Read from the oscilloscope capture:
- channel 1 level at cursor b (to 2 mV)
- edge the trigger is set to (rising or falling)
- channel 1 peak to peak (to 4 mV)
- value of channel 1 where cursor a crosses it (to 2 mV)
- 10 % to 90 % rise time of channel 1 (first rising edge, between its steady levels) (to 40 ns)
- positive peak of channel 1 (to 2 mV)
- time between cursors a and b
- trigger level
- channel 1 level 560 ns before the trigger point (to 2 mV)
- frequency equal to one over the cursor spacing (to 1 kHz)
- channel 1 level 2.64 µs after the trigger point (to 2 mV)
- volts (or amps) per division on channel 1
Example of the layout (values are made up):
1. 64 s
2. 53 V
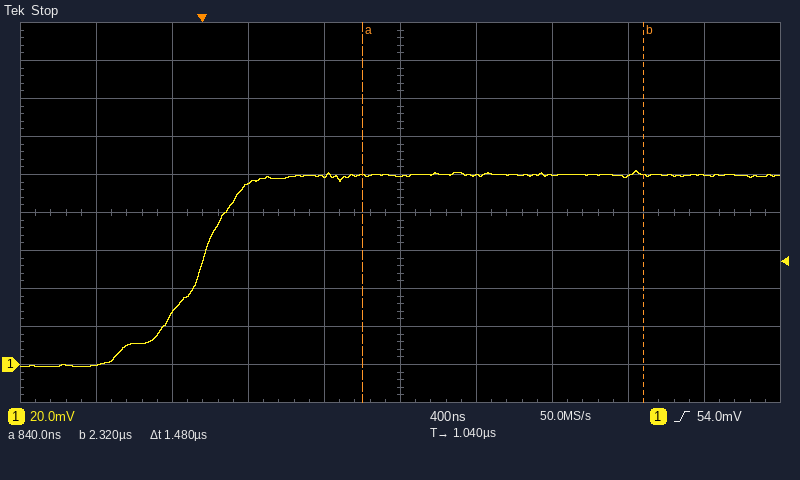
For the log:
1. 100 mV
2. rising
3. 104 mV
4. 100 mV
5. 600 ns
6. 102 mV
7. 1.48 µs
8. 54.0 mV
9. 0 mV
10. 676 kHz
11. 100 mV
12. 20 mV
